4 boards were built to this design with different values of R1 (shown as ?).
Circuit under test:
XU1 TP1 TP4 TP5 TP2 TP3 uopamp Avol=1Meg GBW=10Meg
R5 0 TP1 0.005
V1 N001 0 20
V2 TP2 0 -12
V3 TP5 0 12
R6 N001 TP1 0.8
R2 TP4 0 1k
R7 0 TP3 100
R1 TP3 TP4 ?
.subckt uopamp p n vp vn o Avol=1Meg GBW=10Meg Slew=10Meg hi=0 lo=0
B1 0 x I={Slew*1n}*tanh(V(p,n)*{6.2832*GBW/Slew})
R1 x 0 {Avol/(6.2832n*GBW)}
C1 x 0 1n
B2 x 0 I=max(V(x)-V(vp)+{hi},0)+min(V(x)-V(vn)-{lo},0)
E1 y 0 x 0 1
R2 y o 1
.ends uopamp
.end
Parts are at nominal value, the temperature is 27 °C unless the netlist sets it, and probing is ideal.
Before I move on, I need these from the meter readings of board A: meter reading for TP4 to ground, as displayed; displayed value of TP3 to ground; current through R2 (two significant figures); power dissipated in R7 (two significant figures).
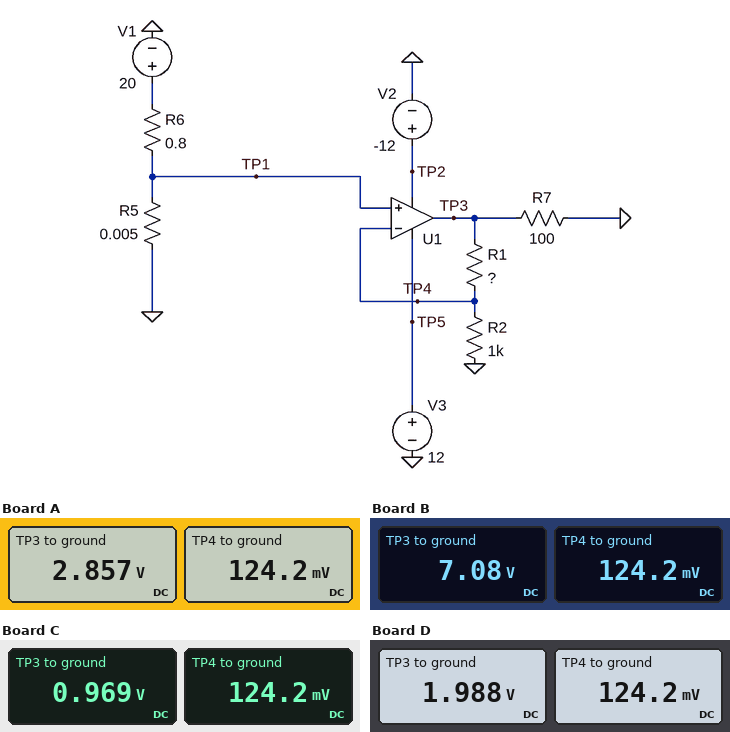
124.2 mV
2.857 V
120 µA
82 mW
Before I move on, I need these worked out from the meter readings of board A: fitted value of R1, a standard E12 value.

22 kΩ
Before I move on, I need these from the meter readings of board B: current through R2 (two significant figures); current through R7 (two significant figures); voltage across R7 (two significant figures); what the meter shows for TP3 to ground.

120 µA
71 mA
7.1 V
7.08 V
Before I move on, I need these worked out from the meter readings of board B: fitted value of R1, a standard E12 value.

56 kΩ
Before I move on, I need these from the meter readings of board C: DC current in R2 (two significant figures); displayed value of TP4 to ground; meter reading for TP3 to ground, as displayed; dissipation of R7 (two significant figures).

120 µA
124.2 mV
0.969 V
9.4 mW
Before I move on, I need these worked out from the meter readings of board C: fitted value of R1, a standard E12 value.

6.8 kΩ
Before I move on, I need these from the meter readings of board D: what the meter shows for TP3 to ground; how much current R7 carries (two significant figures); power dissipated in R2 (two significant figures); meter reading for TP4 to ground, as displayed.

1.988 V
20 mA
15 µW
124.2 mV
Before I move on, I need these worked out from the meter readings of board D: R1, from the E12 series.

15 kΩ
